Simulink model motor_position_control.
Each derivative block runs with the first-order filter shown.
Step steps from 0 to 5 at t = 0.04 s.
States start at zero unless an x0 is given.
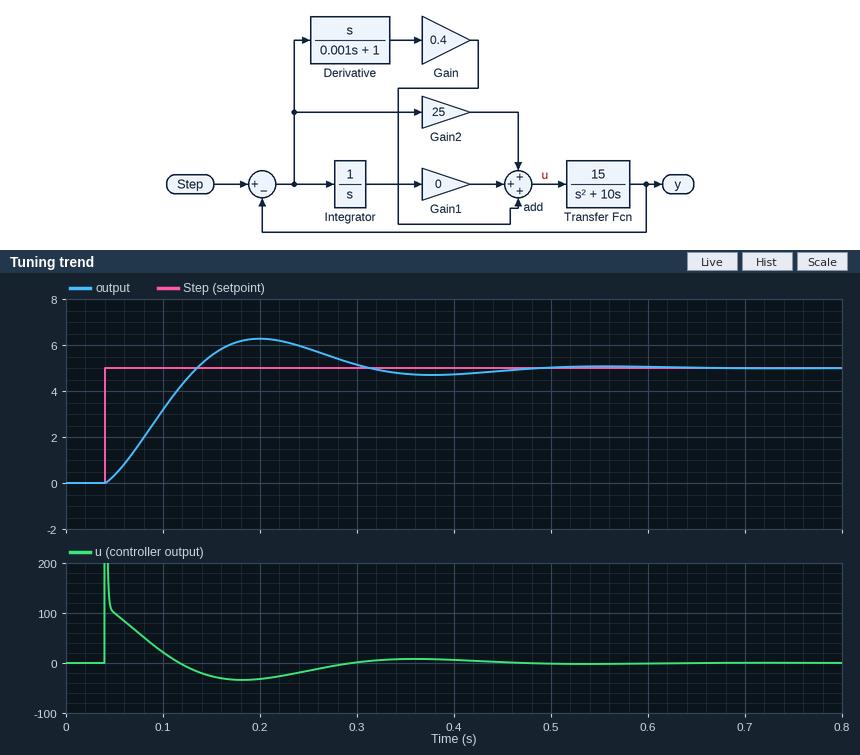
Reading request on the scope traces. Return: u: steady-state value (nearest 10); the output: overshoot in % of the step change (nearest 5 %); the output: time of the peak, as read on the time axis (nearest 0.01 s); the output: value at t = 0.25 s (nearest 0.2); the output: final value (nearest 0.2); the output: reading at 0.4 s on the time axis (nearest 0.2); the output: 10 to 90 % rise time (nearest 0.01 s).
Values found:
0
25 %
0.20 s
5.8
5.0
4.8
0.07 s
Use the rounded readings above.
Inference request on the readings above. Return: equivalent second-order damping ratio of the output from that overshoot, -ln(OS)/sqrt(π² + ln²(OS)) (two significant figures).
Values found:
0.40
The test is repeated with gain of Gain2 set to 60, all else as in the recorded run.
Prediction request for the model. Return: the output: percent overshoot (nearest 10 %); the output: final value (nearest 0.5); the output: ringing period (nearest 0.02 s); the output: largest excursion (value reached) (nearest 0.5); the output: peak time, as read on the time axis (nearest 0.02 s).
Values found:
40 %
5.0
0.22 s
7.0
0.14 s
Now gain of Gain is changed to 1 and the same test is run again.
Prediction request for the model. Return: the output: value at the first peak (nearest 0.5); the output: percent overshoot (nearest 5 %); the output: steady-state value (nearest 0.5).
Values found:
5.5
10 %
5.0
